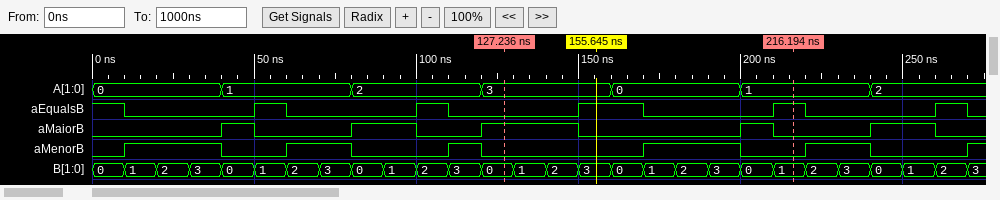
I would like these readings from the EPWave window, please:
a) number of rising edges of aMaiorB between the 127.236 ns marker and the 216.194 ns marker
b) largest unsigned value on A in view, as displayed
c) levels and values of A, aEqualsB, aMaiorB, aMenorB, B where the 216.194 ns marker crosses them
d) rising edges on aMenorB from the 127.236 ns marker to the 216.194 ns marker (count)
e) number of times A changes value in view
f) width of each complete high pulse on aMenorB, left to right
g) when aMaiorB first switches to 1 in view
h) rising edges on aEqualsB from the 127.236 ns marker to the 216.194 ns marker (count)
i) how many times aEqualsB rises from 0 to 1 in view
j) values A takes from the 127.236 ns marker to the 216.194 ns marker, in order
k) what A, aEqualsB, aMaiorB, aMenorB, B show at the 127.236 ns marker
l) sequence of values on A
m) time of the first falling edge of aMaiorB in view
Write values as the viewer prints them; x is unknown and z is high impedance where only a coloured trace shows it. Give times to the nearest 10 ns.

1
3
A=1, aEqualsB=1, aMaiorB=0, aMenorB=0, B=1
1
6
30 ns, 20 ns, 10 ns, 30 ns, 20 ns
40 ns
2
5
3, 0, 1
A=3, aEqualsB=0, aMaiorB=1, aMenorB=0, B=0
0, 1, 2, 3, 0, 1, 2
50 ns
